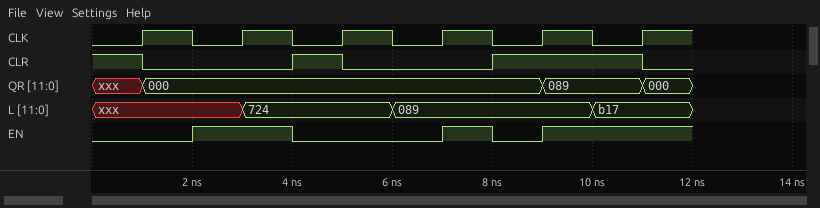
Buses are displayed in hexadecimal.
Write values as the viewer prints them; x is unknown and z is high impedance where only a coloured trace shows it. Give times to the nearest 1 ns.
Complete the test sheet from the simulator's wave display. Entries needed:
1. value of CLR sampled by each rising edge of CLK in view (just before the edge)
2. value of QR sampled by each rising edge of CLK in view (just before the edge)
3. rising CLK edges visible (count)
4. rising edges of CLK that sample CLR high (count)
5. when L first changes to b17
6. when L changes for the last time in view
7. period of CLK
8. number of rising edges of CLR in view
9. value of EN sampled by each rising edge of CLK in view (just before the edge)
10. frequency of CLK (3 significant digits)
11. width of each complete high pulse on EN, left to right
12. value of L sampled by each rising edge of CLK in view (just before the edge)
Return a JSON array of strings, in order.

["1 0 1 0 1 1", "xxx, 000, 000, 000, 000, 089", "6", "4", "10 ns", "10 ns", "2 ns", "2", "0 1 0 0 0 1", "500 MHz", "2 ns, 1 ns", "xxx, xxx, 724, 089, 089, b17"]
